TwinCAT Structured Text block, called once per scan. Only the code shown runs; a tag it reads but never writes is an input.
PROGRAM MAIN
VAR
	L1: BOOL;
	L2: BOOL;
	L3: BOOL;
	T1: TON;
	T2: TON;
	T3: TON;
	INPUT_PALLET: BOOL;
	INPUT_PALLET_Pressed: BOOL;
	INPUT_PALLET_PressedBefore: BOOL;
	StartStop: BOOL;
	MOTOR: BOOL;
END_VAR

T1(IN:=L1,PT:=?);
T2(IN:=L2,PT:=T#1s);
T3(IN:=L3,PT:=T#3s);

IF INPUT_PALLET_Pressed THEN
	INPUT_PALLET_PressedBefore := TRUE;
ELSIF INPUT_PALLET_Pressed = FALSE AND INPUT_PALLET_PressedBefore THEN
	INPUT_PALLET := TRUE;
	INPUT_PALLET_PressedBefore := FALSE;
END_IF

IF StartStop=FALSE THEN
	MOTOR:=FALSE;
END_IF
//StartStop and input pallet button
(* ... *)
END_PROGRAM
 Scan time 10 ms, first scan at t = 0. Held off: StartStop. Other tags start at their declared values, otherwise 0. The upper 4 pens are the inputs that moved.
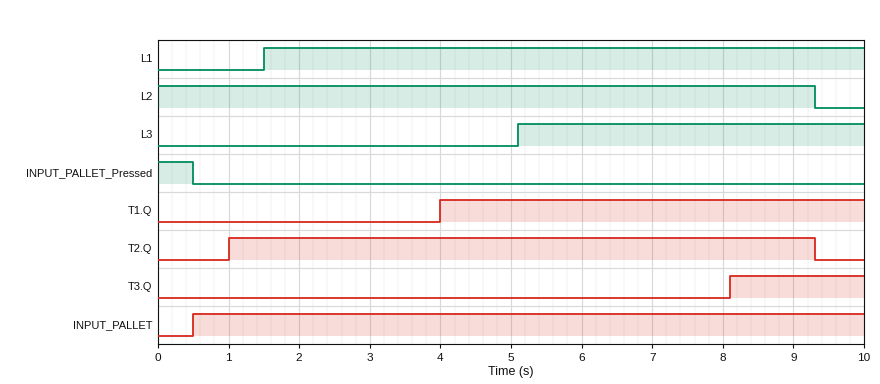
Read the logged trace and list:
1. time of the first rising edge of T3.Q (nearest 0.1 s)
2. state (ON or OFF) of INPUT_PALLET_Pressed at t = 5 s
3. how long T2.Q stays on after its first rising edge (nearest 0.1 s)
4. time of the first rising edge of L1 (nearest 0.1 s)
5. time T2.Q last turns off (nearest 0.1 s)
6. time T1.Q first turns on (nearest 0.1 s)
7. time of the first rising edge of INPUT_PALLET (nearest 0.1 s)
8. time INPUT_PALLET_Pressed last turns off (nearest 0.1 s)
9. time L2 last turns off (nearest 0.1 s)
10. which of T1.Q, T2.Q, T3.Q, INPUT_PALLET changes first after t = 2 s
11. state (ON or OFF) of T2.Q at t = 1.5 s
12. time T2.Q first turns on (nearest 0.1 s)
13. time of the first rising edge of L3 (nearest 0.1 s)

8.1 s
OFF
8.3 s
1.5 s
9.3 s
4.0 s
0.5 s
0.5 s
9.3 s
T1.Q
ON
1.0 s
5.1 s
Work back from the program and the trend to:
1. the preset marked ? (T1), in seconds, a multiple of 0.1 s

2.5 s
